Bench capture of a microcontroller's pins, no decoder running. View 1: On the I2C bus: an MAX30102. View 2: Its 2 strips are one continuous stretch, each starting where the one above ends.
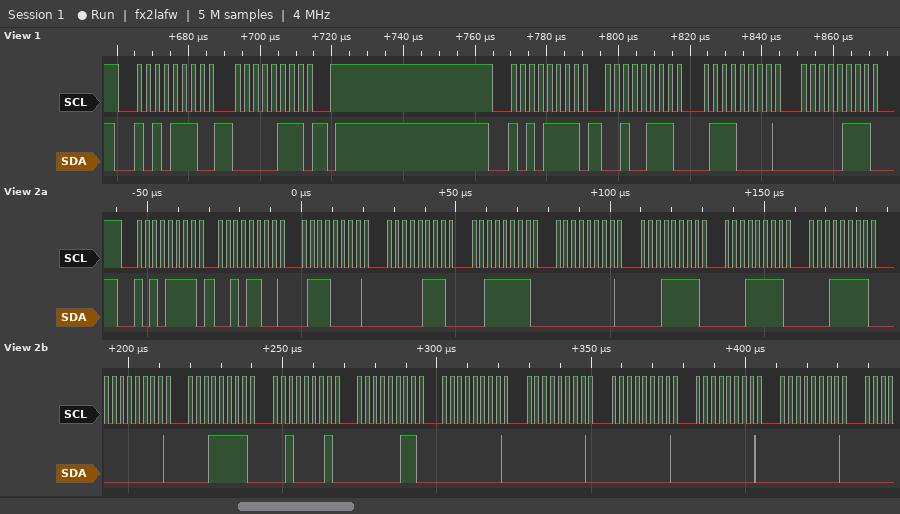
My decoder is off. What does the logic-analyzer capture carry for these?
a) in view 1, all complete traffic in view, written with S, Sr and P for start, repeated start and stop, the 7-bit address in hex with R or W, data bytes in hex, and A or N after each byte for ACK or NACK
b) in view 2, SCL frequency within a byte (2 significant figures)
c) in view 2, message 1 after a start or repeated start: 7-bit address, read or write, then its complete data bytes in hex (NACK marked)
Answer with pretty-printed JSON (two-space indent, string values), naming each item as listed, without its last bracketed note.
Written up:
{
  "in view 1, all complete traffic in view, written with S, Sr and P for start, repeated start and stop, the 7-bit address in hex with R or W, data bytes in hex, and A or N after each byte for ACK or NACK": "S 57W A 07 A P S 57R A 27 A 70 A 07 A",
  "in view 2, SCL frequency within a byte": "400 kHz",
  "in view 2, message 1 after a start or repeated start: 7-bit address, read or write, then its complete data bytes in hex": "0x57 read: 2C 70 07 3F 00 1F 1F 1F 00 1F 21 03 00 00 00 00 00"
}
